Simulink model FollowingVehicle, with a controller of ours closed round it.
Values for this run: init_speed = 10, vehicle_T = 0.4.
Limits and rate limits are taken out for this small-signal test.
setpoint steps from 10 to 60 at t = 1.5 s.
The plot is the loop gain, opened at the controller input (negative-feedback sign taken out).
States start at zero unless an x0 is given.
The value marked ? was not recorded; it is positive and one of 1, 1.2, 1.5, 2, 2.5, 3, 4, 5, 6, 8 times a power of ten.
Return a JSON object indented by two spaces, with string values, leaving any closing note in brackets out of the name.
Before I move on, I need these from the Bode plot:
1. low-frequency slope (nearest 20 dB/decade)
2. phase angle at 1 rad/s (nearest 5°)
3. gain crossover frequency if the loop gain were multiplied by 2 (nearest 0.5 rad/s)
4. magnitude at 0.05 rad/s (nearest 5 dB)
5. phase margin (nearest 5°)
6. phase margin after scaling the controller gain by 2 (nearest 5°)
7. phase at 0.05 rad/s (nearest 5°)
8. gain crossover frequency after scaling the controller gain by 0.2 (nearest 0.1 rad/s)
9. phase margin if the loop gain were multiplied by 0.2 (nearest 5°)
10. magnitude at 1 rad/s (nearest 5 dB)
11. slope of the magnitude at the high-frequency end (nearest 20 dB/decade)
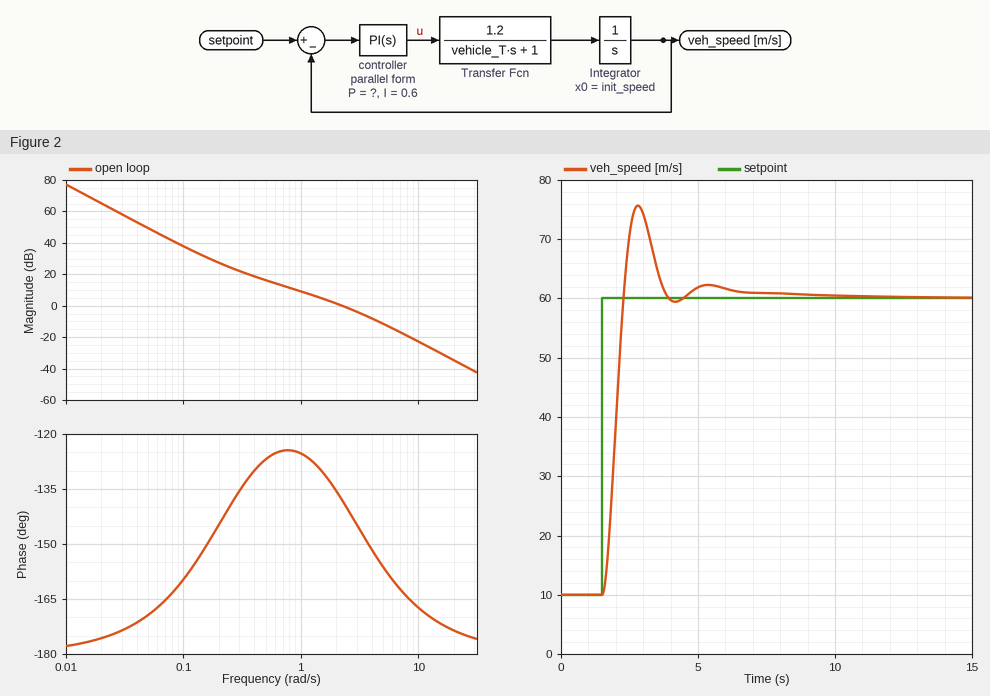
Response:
{
  "low-frequency slope": "-40 dB/decade",
  "phase angle at 1 rad/s": "-125°",
  "gain crossover frequency if the loop gain were multiplied by 2": "3.5 rad/s",
  "magnitude at 0.05 rad/s": "50 dB",
  "phase margin": "40°",
  "phase margin after scaling the controller gain by 2": "30°",
  "phase at 0.05 rad/s": "-170°",
  "gain crossover frequency after scaling the controller gain by 0.2": "0.6 rad/s",
  "phase margin if the loop gain were multiplied by 0.2": "55°",
  "magnitude at 1 rad/s": "10 dB",
  "slope of the magnitude at the high-frequency end": "-40 dB/decade"
}
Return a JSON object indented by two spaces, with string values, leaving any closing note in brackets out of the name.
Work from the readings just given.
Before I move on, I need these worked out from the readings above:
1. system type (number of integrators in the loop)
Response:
{
  "system type": "2"
}
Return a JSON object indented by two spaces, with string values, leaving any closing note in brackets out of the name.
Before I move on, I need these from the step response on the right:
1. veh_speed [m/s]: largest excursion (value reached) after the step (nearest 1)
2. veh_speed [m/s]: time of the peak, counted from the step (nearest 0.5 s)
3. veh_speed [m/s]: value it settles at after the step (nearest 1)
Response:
{
  "veh_speed [m/s]: largest excursion (value reached) after the step": "76",
  "veh_speed [m/s]: time of the peak, counted from the step": "1.5 s",
  "veh_speed [m/s]: value it settles at after the step": "60"
}
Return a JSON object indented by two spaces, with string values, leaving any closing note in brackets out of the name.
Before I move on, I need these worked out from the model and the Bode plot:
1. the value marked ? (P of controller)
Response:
{
  "the value marked ?": "2.5"
}
